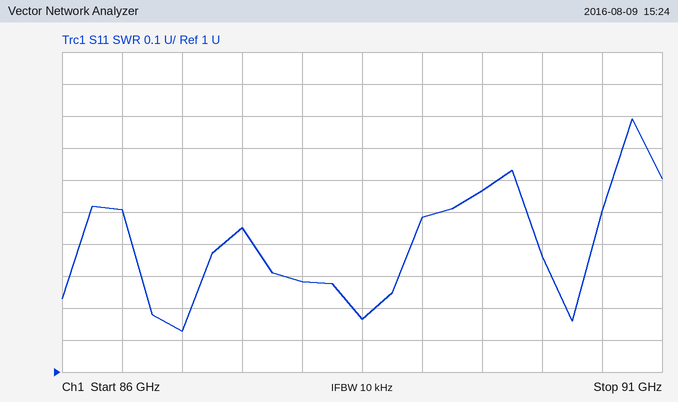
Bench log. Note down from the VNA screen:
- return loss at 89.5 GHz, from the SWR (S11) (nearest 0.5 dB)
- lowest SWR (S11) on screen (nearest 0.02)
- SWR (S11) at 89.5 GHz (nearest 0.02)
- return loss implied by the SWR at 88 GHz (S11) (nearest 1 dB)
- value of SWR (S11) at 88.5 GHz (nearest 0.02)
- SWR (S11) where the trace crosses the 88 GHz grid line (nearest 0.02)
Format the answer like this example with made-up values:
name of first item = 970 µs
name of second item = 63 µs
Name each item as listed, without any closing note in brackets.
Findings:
return loss at 89.5 GHz, from the SWR (S11) = 13.0 dB
lowest SWR (S11) on screen = 1.12
SWR (S11) at 89.5 GHz = 1.56
return loss implied by the SWR at 88 GHz (S11) = 18 dB
value of SWR (S11) at 88.5 GHz = 1.16
SWR (S11) where the trace crosses the 88 GHz grid line = 1.28
